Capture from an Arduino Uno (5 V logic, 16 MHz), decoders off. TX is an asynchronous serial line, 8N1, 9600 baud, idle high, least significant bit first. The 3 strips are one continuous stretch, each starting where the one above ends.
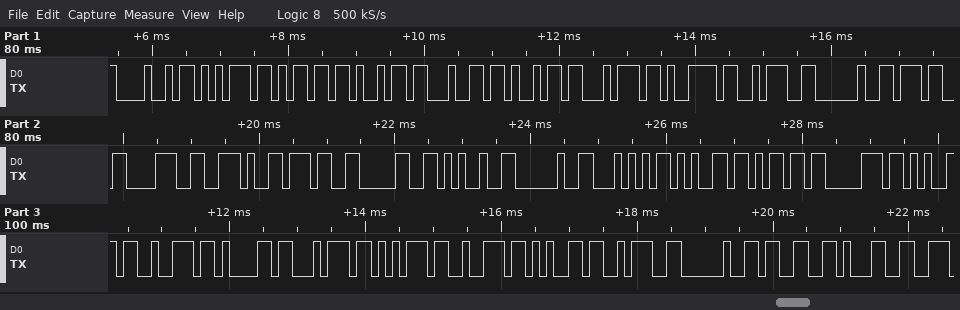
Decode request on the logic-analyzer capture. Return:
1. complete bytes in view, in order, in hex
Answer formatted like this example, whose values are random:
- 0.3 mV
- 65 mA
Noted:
- 48 75 6D 69 64 69 74 79 3A 20 37 38 2E 37 30 25 20 54 65 6D 70 65 72 61 74 75 72 65 3A 20 33 31
